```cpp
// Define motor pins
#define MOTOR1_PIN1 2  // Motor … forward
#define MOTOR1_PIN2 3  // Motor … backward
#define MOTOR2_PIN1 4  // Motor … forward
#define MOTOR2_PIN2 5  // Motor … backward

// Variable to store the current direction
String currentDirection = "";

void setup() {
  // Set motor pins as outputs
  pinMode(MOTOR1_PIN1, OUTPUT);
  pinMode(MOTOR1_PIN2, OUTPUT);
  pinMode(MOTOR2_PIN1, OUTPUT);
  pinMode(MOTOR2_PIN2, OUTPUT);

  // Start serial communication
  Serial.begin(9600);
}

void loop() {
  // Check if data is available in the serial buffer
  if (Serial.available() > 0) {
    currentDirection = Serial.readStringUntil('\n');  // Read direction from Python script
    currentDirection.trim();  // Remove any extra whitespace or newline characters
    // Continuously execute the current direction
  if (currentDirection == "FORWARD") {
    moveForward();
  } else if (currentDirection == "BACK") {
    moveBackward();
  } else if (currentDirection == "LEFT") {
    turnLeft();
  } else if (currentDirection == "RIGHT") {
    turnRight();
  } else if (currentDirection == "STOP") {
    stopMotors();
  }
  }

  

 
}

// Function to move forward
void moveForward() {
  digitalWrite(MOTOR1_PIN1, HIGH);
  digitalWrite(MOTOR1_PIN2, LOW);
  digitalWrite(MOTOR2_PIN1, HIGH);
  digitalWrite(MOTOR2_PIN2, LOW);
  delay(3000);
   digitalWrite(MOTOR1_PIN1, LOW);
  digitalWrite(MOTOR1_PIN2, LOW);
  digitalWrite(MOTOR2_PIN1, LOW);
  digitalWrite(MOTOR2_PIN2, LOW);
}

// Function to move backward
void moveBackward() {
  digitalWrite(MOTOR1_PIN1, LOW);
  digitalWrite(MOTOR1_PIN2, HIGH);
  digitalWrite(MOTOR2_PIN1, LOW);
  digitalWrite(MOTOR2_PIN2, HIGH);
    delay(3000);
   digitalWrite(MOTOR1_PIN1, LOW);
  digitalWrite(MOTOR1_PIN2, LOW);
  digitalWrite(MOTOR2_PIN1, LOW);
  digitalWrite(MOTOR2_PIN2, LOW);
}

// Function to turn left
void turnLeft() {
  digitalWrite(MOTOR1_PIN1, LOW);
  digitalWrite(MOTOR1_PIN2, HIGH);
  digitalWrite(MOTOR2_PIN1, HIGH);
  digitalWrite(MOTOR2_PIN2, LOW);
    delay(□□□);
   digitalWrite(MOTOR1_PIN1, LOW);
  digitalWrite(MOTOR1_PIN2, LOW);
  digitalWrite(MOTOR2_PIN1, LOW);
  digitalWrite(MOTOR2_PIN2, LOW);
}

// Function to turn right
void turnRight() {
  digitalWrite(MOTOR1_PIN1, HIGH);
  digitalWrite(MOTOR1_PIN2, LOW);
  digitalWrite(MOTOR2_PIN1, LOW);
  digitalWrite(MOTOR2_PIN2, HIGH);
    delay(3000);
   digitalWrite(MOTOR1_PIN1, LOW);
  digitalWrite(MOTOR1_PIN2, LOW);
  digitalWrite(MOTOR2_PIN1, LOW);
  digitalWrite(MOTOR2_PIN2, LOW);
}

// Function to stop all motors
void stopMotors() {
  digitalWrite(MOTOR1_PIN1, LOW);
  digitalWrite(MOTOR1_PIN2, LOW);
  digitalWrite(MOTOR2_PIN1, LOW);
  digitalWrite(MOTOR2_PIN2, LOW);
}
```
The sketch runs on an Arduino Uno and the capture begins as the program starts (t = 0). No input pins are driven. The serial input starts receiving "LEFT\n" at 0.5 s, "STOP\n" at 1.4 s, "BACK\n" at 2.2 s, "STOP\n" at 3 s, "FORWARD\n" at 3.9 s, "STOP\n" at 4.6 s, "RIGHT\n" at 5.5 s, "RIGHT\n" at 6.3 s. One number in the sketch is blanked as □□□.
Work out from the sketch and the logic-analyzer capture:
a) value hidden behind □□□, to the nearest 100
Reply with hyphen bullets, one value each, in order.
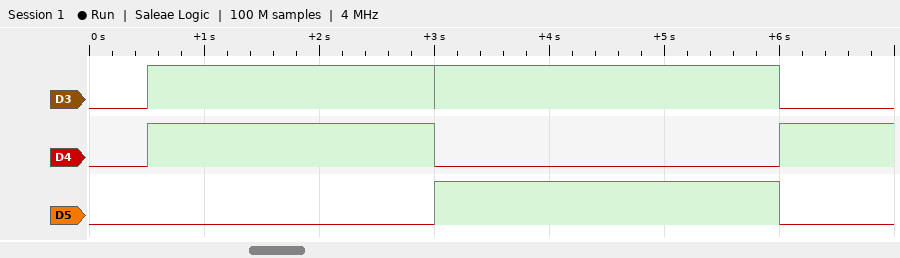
- 2500
